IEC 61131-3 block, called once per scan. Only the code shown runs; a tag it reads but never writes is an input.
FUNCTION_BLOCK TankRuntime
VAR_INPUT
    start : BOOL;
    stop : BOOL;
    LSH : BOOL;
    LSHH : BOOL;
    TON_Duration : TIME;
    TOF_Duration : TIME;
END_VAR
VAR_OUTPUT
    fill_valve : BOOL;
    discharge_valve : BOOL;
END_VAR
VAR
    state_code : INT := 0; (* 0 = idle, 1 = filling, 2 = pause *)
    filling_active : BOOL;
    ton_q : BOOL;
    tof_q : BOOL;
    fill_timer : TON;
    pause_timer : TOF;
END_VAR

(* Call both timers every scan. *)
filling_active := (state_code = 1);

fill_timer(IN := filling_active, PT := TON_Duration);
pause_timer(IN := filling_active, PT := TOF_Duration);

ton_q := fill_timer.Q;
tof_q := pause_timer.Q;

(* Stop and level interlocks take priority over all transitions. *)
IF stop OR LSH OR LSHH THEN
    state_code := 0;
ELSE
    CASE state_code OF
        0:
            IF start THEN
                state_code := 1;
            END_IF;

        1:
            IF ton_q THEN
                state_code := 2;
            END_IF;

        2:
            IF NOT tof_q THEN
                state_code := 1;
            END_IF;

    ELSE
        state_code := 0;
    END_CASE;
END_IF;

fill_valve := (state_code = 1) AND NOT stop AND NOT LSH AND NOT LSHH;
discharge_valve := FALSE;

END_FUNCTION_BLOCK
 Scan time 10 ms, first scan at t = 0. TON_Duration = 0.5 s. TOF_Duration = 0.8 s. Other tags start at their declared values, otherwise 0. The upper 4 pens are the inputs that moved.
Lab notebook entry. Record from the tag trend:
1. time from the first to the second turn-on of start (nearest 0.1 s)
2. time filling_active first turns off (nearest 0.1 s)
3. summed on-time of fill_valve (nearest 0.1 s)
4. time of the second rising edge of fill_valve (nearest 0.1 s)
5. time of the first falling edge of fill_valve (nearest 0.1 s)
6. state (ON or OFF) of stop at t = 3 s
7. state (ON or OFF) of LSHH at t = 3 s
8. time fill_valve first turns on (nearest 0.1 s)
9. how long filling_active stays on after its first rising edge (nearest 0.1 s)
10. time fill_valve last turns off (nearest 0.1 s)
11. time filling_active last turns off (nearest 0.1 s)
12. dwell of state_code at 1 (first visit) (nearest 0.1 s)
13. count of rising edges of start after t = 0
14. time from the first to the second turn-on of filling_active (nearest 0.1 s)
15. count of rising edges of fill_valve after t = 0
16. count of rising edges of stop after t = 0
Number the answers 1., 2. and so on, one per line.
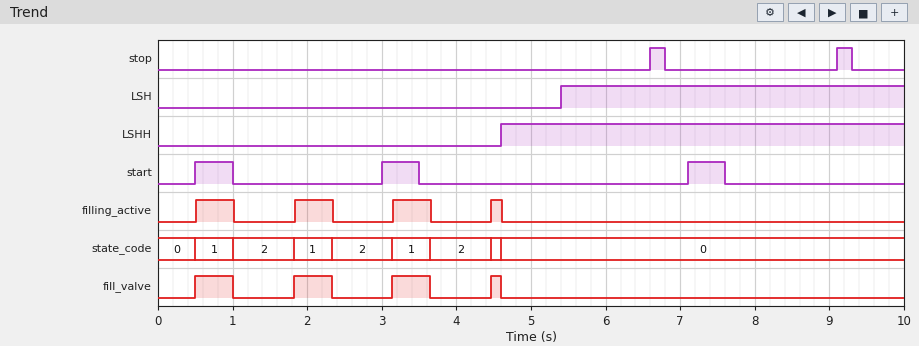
1. 2.5 s
2. 1.0 s
3. 1.7 s
4. 1.8 s
5. 1.0 s
6. OFF
7. OFF
8. 0.5 s
9. 0.5 s
10. 4.6 s
11. 4.6 s
12. 0.5 s
13. 3
14. 1.3 s
15. 4
16. 2
